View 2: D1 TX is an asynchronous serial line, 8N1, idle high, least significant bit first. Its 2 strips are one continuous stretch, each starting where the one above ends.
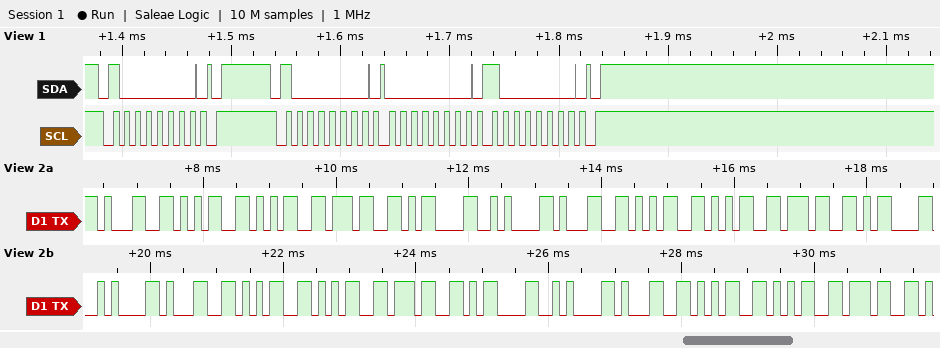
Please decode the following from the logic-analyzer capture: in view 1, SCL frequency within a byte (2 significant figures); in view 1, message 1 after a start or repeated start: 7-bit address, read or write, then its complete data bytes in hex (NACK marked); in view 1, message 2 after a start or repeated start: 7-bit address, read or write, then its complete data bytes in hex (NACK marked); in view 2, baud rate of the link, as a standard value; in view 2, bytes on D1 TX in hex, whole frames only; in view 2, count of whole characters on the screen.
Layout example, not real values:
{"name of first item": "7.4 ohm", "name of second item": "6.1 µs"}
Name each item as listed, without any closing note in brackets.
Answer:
{"in view 1, SCL frequency within a byte": "100 kHz", "in view 1, message 1 after a start or repeated start: 7-bit address, read or write, then its complete data bytes in hex": "0x40 write", "in view 1, message 2 after a start or repeated start: 7-bit address, read or write, then its complete data bytes in hex": "0x40 write: 00 80", "in view 2, baud rate of the link, as a standard value": "9600 baud", "in view 2, bytes on D1 TX in hex, whole frames only": "0x31 0x35 0x35 0x37 0x0D 0x0A 0x31 0x35 0x35 0x37 0x0D 0x0A 0x31 0x35 0x35 0x37 0x0D 0x0A 0x31 0x35 0x35 0x37", "in view 2, count of whole characters on the screen": "22"}
